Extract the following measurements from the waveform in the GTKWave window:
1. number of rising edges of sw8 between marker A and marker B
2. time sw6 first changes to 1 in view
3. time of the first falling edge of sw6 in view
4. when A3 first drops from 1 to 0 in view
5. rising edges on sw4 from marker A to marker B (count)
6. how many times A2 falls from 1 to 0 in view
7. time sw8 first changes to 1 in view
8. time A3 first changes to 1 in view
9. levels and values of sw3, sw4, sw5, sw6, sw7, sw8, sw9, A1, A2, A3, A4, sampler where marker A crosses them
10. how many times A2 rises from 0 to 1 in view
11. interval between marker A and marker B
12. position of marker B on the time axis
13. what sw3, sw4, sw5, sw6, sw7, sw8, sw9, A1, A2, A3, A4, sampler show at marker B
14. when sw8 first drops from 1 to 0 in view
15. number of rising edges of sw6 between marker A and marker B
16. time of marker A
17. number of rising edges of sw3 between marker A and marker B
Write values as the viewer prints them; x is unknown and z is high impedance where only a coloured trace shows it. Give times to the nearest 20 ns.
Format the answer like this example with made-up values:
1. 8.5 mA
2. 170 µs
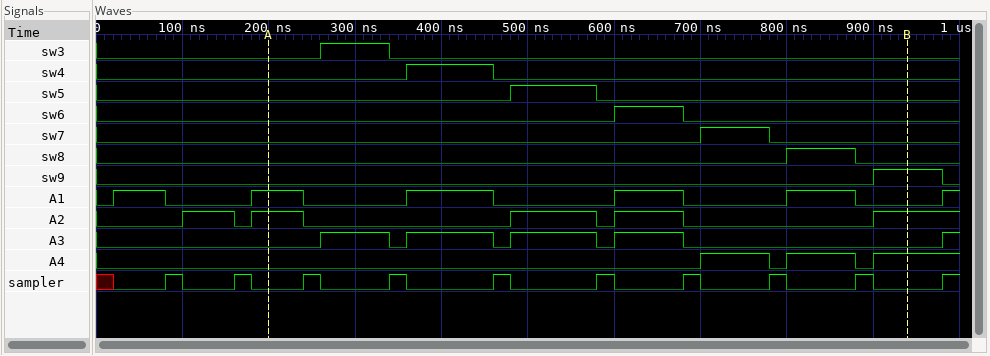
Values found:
1. 1
2. 600 ns
3. 680 ns
4. 340 ns
5. 1
6. 4
7. 800 ns
8. 260 ns
9. sw3=0, sw4=0, sw5=0, sw6=0, sw7=0, sw8=0, sw9=0, A1=1, A2=1, A3=0, A4=0, sampler=0
10. 5
11. 740 ns
12. 940 ns
13. sw3=0, sw4=0, sw5=0, sw6=0, sw7=0, sw8=0, sw9=1, A1=0, A2=1, A3=0, A4=1, sampler=0
14. 880 ns
15. 1
16. 200 ns
17. 1
